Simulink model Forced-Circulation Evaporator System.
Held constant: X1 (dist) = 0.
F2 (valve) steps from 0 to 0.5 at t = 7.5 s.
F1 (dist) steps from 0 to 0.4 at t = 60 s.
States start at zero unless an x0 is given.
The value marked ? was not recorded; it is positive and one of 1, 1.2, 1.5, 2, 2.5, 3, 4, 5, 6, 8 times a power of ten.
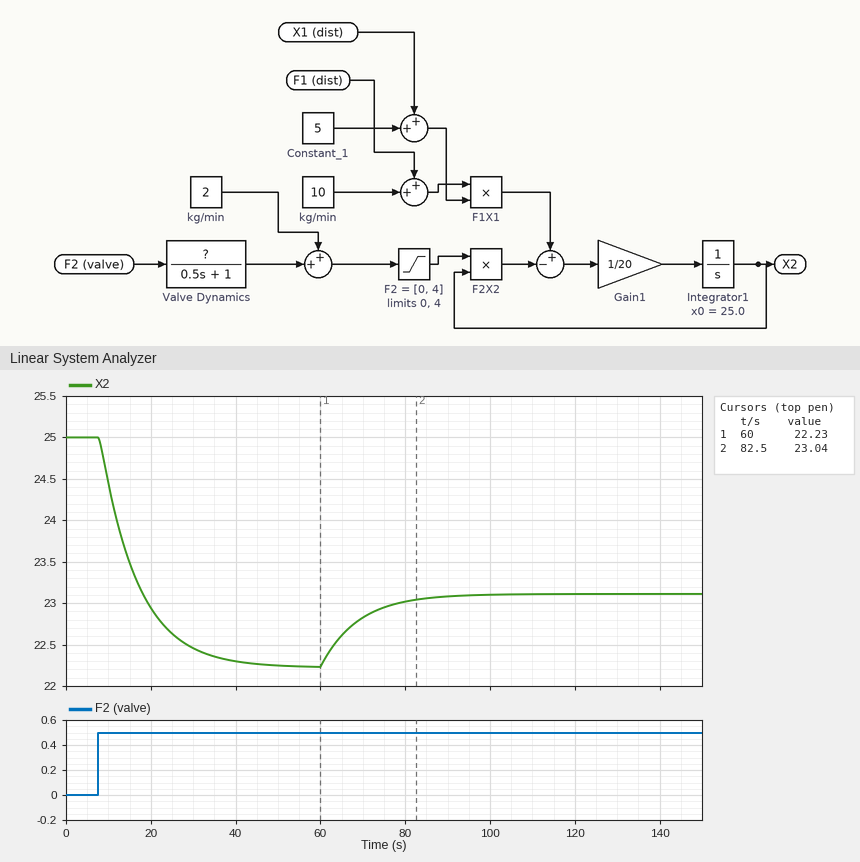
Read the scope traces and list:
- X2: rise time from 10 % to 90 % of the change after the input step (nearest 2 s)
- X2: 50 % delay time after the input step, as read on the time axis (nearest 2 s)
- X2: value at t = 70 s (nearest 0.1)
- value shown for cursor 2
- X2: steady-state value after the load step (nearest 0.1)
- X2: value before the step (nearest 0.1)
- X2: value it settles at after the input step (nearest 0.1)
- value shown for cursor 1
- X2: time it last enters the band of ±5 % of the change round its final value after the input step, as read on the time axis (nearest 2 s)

20 s
14 s
22.8
23.04
23.1
25.0
22.2
22.23
34 s
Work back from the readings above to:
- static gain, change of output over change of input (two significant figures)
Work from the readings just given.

-5.6
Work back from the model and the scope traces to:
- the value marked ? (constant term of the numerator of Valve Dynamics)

0.5
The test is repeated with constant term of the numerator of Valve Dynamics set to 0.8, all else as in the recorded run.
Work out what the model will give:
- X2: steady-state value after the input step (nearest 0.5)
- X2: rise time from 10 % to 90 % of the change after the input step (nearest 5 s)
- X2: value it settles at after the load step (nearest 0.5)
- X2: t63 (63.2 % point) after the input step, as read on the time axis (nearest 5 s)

21.0
20 s
21.5
15 s
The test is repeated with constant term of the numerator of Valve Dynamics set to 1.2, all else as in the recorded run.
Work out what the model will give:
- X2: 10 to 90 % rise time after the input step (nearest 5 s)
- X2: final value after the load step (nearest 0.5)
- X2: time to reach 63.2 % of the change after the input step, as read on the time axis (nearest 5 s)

15 s
20.0
15 s
